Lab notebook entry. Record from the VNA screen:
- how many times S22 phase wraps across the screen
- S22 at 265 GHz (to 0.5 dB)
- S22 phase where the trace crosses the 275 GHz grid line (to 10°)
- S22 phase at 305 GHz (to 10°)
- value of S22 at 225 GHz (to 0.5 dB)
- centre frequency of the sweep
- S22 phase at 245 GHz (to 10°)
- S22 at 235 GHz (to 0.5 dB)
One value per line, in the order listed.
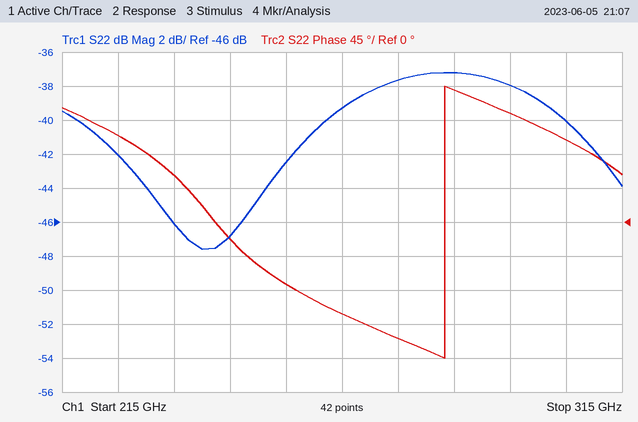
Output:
1
-39.5 dB
-150°
110°
-42.0 dB
265 GHz
-20°
-46.0 dB
